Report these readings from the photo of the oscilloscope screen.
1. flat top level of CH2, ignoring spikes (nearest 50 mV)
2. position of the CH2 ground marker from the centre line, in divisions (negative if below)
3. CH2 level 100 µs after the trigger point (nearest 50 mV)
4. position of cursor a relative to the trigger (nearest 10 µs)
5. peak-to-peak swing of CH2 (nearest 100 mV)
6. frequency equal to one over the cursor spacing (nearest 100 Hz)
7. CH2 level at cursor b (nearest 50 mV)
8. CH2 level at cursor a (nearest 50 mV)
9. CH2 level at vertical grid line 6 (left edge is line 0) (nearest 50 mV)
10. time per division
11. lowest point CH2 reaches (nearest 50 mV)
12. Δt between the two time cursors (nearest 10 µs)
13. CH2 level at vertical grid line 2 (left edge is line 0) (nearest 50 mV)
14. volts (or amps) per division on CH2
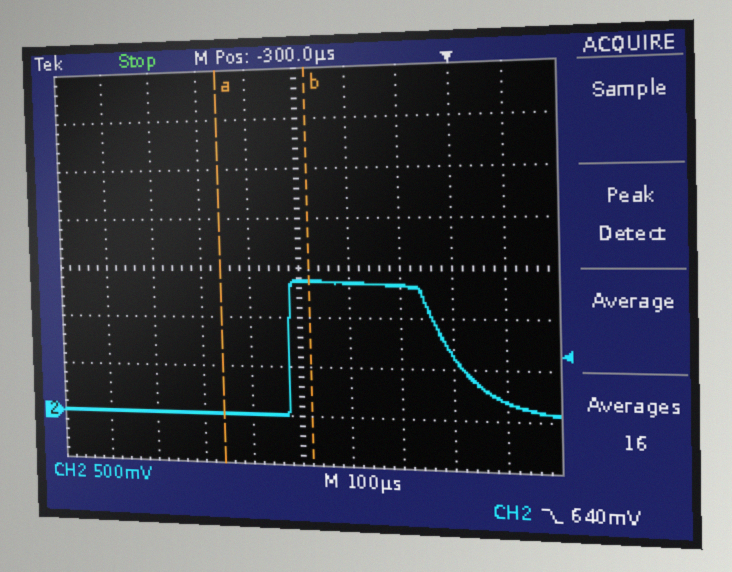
1.35 V
-3.0 div
200 mV
-460 µs
1.40 V
5.6 kHz
1.35 V
0 mV
1.35 V
100 µs
0 mV
180 µs
0 mV
500 mV
